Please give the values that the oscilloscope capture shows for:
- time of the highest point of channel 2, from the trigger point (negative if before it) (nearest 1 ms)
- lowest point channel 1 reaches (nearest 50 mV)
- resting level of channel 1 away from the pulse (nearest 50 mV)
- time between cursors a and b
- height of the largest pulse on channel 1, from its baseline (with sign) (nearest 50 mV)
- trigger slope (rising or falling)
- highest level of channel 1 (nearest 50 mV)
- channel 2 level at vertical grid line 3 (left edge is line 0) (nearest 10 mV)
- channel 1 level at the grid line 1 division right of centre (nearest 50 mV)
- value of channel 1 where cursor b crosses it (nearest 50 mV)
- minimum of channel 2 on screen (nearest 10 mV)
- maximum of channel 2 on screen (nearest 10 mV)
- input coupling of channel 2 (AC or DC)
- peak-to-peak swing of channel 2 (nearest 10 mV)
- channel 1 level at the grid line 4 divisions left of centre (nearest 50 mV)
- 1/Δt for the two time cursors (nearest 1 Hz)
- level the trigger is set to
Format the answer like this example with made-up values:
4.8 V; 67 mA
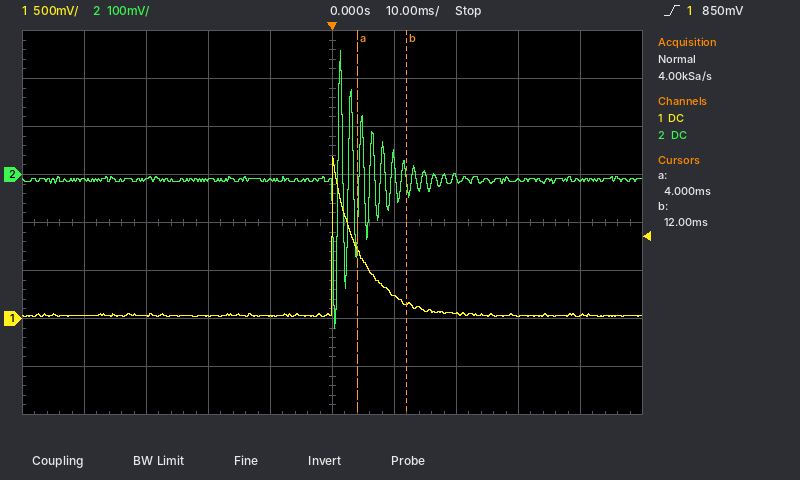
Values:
+1 ms; 0 mV; 50 mV; 8 ms; +1.65 V; rising; 1.70 V; -10 mV; 250 mV; 150 mV; -320 mV; 260 mV; DC; 580 mV; 50 mV; 125 Hz; 850 mV
